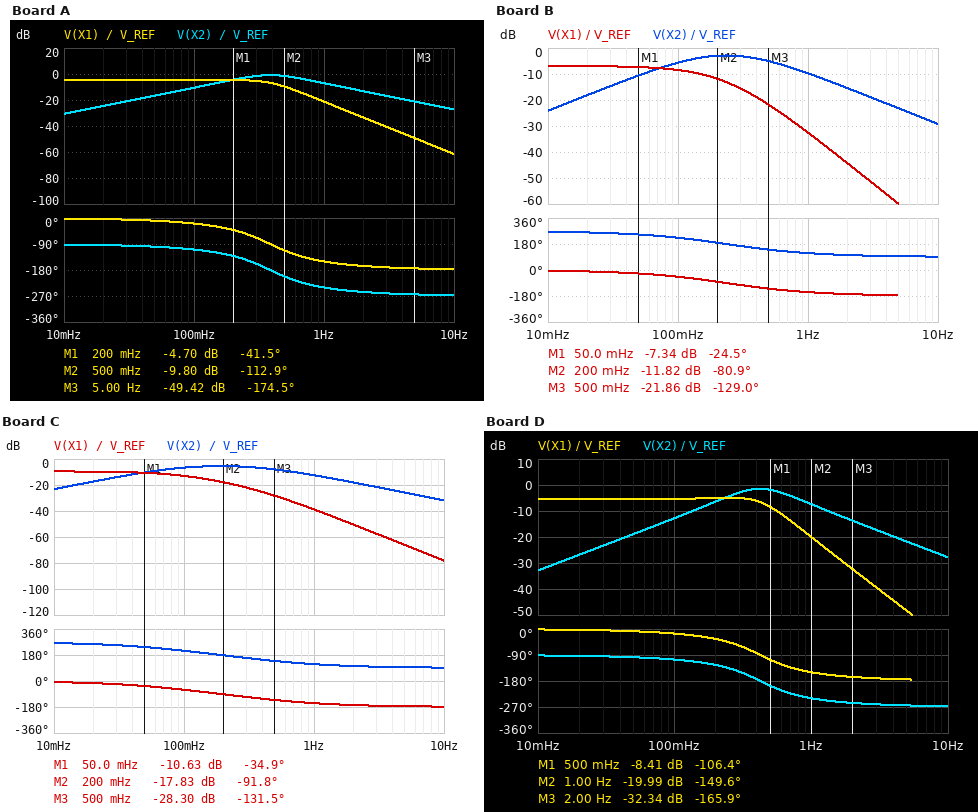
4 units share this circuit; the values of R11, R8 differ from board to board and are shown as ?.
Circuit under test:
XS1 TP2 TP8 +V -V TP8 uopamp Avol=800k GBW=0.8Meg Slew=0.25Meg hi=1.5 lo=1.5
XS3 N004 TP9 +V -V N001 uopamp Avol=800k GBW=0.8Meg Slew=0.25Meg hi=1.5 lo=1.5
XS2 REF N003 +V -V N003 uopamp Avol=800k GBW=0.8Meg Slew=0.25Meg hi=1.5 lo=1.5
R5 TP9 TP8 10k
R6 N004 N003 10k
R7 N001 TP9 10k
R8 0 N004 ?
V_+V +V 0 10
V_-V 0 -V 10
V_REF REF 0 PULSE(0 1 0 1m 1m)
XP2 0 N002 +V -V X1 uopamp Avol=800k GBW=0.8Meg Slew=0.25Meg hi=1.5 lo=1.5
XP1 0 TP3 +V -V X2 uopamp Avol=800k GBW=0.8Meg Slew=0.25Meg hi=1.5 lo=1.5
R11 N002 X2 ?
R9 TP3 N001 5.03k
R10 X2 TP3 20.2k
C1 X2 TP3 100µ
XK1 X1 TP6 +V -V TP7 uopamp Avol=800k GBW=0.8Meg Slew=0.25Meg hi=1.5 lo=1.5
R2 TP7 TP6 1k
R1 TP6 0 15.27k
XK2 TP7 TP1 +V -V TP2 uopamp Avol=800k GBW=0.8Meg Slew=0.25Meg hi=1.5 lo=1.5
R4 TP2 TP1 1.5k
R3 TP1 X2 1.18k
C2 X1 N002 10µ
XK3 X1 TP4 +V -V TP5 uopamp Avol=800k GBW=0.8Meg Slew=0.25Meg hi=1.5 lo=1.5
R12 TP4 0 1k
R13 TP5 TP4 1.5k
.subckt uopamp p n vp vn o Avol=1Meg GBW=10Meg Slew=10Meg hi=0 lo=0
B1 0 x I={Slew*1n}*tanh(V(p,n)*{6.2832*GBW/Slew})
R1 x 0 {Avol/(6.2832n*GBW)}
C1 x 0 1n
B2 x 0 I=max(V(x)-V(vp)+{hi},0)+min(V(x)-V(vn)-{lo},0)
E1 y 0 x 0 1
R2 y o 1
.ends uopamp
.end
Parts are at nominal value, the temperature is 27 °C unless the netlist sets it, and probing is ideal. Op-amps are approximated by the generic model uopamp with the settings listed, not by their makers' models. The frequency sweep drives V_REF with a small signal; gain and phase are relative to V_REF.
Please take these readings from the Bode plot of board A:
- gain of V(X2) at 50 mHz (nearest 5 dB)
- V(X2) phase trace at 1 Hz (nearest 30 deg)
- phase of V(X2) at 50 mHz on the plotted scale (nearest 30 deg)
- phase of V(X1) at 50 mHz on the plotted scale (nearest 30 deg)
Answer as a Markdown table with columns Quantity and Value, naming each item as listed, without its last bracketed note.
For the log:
| Quantity | Value |
|---|---|
| gain of V(X2) at 50 mHz | -15 dB |
| V(X2) phase trace at 1 Hz | -240 deg |
| phase of V(X2) at 50 mHz on the plotted scale | -90 deg |
| phase of V(X1) at 50 mHz on the plotted scale | 0 deg |
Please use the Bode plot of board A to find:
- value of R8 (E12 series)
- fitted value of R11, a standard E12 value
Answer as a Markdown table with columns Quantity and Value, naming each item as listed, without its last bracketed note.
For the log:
| Quantity | Value |
|---|---|
| value of R8 | 22 kΩ |
| fitted value of R11, a standard E12 value | 82 kΩ |
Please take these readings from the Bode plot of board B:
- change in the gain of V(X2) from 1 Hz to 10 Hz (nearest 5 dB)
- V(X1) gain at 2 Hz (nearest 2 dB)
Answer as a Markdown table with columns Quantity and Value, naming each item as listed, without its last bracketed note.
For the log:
| Quantity | Value |
|---|---|
| change in the gain of V(X2) from 1 Hz to 10 Hz | -20 dB |
| V(X1) gain at 2 Hz | -44 dB |
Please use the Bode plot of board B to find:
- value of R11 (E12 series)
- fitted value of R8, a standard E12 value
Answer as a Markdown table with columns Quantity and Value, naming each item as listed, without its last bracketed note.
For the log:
| Quantity | Value |
|---|---|
| value of R11 | 220 kΩ |
| fitted value of R8, a standard E12 value | 12 kΩ |
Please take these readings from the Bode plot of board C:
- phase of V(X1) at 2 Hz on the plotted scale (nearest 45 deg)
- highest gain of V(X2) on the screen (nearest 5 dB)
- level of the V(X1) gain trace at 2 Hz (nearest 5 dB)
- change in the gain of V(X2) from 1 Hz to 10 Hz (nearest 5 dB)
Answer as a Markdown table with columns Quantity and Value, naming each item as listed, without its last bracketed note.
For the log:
| Quantity | Value |
|---|---|
| phase of V(X1) at 2 Hz on the plotted scale | -180 deg |
| highest gain of V(X2) on the screen | -5 dB |
| level of the V(X1) gain trace at 2 Hz | -50 dB |
| change in the gain of V(X2) from 1 Hz to 10 Hz | -20 dB |
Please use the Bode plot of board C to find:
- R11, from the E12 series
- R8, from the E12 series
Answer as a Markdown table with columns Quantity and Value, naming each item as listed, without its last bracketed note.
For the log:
| Quantity | Value |
|---|---|
| R11, from the E12 series | 330 kΩ |
| R8, from the E12 series | 6.8 kΩ |
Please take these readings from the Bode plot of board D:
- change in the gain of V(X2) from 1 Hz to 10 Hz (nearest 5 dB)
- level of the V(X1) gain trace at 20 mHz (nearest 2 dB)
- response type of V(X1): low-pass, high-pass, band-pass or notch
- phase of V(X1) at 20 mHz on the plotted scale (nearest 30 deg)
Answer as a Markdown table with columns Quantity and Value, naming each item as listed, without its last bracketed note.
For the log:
| Quantity | Value |
|---|---|
| change in the gain of V(X2) from 1 Hz to 10 Hz | -20 dB |
| level of the V(X1) gain trace at 20 mHz | -6 dB |
| response type of V(X1): low-pass, high-pass, band-pass or notch | low-pass |
| phase of V(X1) at 20 mHz on the plotted scale | 0 deg |
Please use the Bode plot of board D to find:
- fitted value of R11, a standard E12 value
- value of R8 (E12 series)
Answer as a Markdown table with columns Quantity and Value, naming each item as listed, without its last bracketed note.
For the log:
| Quantity | Value |
|---|---|
| fitted value of R11, a standard E12 value | 68 kΩ |
| value of R8 | 18 kΩ |
